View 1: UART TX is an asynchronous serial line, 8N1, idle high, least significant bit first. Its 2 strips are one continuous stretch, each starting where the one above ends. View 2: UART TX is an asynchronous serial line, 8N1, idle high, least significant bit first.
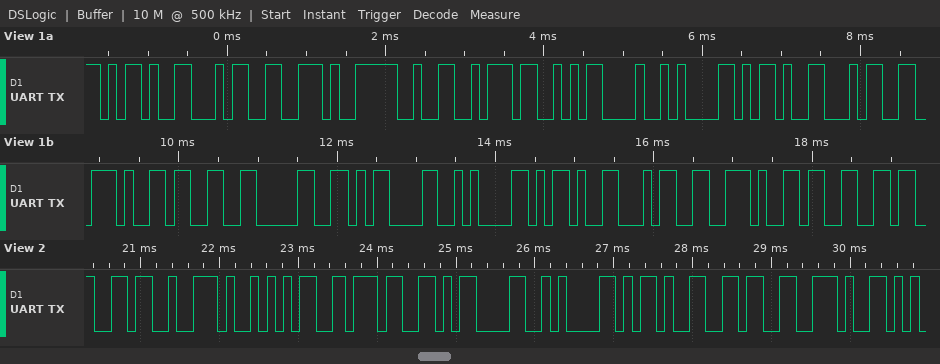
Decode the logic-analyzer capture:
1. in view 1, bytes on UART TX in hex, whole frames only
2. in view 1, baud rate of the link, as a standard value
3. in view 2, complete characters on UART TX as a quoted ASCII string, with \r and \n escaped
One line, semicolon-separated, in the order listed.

0x2D 0x34 0x2E 0x32 0x37 0x0D 0x0A 0x2D 0x34 0x2E 0x33 0x30 0x0D 0x0A 0x2D 0x34 0x2E 0x33; 9600 baud; "6.57\r\n-6."
